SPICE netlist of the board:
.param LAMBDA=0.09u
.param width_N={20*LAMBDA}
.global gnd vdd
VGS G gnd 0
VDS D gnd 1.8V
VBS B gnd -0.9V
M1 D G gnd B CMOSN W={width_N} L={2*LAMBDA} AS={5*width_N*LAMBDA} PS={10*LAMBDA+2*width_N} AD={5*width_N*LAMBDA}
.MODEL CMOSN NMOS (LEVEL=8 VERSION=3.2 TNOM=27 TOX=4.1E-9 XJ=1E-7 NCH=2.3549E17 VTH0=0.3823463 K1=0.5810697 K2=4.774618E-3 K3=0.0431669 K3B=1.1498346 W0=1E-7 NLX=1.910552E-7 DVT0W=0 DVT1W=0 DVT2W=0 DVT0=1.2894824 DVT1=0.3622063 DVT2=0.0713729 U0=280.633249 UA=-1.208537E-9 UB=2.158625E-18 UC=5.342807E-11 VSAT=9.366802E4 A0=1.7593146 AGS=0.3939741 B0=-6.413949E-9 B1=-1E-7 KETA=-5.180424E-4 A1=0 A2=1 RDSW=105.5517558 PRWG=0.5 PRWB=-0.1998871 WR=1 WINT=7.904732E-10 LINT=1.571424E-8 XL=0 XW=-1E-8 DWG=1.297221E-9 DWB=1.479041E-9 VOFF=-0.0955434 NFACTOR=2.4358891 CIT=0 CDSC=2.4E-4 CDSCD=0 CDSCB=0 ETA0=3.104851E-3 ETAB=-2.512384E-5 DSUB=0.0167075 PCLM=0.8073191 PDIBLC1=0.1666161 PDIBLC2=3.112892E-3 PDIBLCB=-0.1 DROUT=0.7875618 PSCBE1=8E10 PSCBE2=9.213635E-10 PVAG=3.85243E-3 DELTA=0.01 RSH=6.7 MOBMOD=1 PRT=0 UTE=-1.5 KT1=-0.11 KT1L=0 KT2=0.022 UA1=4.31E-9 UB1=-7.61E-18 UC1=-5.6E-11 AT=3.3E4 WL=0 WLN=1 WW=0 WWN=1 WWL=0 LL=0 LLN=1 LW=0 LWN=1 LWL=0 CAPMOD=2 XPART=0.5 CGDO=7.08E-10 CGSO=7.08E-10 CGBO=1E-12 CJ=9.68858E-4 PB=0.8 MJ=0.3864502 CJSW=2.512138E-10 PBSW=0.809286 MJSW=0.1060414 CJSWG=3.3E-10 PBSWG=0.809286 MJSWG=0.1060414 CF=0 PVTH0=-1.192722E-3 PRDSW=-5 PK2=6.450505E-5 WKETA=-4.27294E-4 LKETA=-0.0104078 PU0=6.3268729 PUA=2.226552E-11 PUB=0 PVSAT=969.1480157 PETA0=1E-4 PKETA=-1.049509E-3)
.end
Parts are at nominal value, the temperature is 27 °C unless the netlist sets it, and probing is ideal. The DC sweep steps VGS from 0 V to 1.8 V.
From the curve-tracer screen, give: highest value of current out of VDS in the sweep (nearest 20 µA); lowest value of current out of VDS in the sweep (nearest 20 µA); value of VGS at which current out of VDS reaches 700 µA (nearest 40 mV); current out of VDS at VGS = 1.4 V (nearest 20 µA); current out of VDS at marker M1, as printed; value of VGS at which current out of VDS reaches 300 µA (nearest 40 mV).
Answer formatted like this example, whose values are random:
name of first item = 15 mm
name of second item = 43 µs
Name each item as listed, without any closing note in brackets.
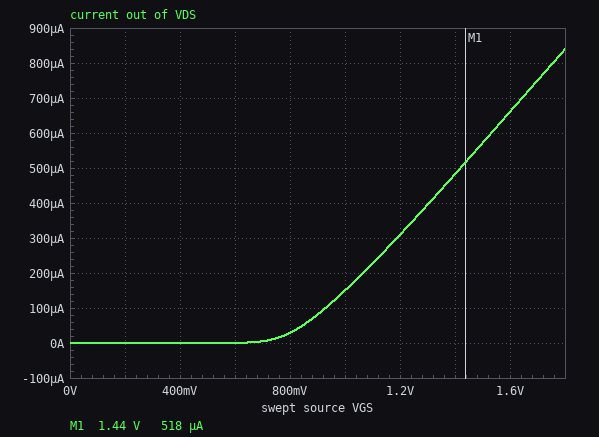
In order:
highest value of current out of VDS in the sweep = 840 µA
lowest value of current out of VDS in the sweep = 0 A
value of VGS at which current out of VDS reaches 700 µA = 1.64 V
current out of VDS at VGS = 1.4 V = 480 µA
current out of VDS at marker M1, as printed = 518 µA
value of VGS at which current out of VDS reaches 300 µA = 1.20 V
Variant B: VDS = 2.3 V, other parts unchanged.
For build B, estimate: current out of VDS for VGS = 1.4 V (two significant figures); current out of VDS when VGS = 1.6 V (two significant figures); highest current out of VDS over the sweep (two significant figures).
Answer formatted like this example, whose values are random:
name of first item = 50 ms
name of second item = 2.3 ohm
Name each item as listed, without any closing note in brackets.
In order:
current out of VDS for VGS = 1.4 V = 500 µA
current out of VDS when VGS = 1.6 V = 680 µA
highest current out of VDS over the sweep = 860 µA
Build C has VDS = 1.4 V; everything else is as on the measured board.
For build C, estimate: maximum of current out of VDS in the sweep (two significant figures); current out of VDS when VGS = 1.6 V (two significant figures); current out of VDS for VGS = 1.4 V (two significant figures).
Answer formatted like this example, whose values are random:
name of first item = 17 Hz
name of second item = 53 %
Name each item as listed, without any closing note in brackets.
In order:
maximum of current out of VDS in the sweep = 820 µA
current out of VDS when VGS = 1.6 V = 640 µA
current out of VDS for VGS = 1.4 V = 470 µA
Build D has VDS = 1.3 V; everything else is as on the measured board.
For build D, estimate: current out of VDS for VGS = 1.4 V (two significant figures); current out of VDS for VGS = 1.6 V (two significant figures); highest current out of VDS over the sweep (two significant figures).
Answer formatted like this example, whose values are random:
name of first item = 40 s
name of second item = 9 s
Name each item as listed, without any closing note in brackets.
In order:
current out of VDS for VGS = 1.4 V = 460 µA
current out of VDS for VGS = 1.6 V = 640 µA
highest current out of VDS over the sweep = 810 µA
